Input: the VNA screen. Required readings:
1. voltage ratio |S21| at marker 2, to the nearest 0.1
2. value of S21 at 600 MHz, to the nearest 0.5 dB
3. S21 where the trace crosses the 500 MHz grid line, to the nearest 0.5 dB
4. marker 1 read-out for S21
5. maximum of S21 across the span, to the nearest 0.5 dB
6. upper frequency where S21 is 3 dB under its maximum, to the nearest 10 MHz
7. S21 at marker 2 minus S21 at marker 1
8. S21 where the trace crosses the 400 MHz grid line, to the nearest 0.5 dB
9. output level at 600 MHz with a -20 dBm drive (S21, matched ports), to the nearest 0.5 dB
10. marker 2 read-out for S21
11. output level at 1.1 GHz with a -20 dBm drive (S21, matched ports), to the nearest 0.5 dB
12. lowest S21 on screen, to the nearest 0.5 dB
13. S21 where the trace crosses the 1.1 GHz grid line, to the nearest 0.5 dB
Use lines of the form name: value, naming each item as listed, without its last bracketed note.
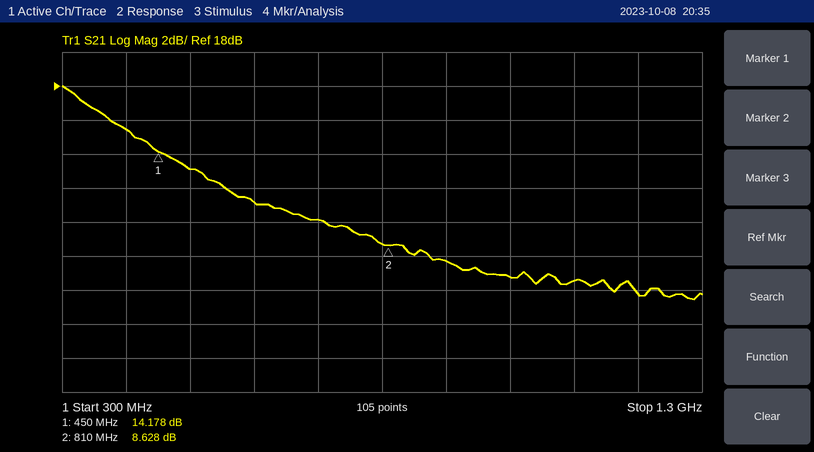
voltage ratio |S21| at marker 2, to the nearest 0.1: 2.7
value of S21 at 600 MHz, to the nearest 0.5 dB: 11.0 dB
S21 where the trace crosses the 500 MHz grid line, to the nearest 0.5 dB: 13.0 dB
marker 1 read-out for S21: 14.178 dB
maximum of S21 across the span, to the nearest 0.5 dB: 18.0 dB
upper frequency where S21 is 3 dB under its maximum, to the nearest 10 MHz: 410 MHz
S21 at marker 2 minus S21 at marker 1: -5.550 dB
S21 where the trace crosses the 400 MHz grid line, to the nearest 0.5 dB: 15.5 dB
output level at 600 MHz with a -20 dBm drive (S21, matched ports), to the nearest 0.5 dB: -9.0 dBm
marker 2 read-out for S21: 8.628 dB
output level at 1.1 GHz with a -20 dBm drive (S21, matched ports), to the nearest 0.5 dB: -13.5 dBm
lowest S21 on screen, to the nearest 0.5 dB: 5.5 dB
S21 where the trace crosses the 1.1 GHz grid line, to the nearest 0.5 dB: 6.5 dB
